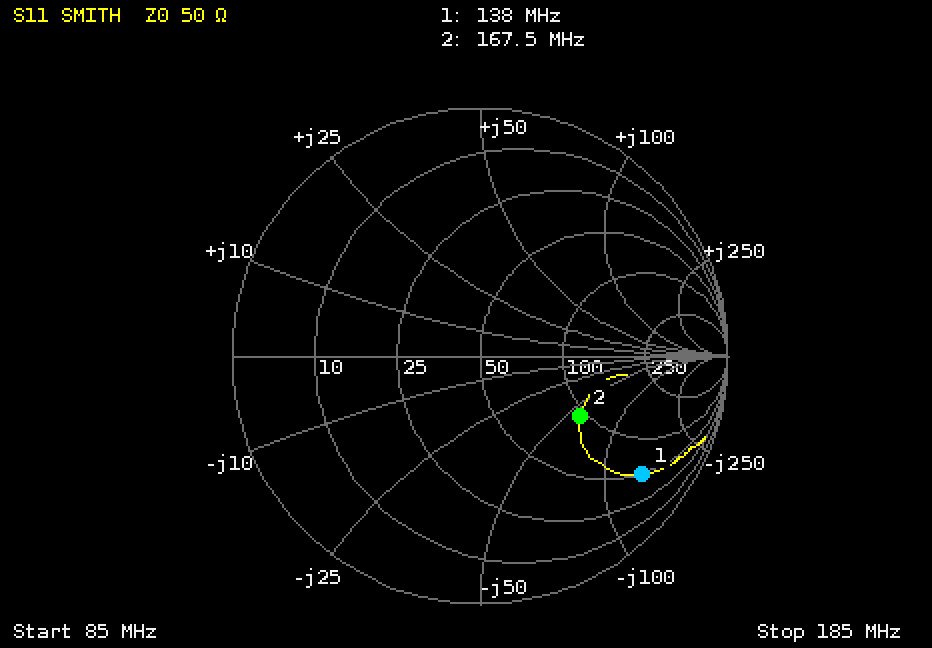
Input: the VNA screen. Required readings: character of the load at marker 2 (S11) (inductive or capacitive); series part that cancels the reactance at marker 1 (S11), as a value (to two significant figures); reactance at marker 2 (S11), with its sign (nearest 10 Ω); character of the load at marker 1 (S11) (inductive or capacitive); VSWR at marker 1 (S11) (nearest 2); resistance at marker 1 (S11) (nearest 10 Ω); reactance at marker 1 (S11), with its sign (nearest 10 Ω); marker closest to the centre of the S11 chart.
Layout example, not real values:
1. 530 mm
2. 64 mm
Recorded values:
1. capacitive
2. 160 nH
3. -60 Ω
4. capacitive
5. 10
6. 50 Ω
7. -140 Ω
8. marker 2
